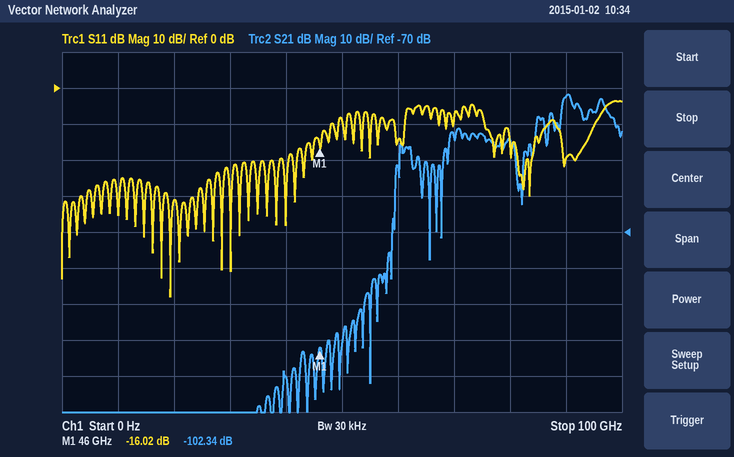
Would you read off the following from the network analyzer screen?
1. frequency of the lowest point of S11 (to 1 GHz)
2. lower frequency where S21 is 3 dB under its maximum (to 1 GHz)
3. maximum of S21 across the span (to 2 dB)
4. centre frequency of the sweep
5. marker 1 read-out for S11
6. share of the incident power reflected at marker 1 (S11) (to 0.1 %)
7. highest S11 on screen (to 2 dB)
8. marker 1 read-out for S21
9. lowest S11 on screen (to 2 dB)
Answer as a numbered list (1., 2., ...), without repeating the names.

1. 19 GHz
2. 89 GHz
3. -32 dB
4. 50 GHz
5. -16.02 dB
6. 2.5 %
7. -4 dB
8. -102.34 dB
9. -58 dB
